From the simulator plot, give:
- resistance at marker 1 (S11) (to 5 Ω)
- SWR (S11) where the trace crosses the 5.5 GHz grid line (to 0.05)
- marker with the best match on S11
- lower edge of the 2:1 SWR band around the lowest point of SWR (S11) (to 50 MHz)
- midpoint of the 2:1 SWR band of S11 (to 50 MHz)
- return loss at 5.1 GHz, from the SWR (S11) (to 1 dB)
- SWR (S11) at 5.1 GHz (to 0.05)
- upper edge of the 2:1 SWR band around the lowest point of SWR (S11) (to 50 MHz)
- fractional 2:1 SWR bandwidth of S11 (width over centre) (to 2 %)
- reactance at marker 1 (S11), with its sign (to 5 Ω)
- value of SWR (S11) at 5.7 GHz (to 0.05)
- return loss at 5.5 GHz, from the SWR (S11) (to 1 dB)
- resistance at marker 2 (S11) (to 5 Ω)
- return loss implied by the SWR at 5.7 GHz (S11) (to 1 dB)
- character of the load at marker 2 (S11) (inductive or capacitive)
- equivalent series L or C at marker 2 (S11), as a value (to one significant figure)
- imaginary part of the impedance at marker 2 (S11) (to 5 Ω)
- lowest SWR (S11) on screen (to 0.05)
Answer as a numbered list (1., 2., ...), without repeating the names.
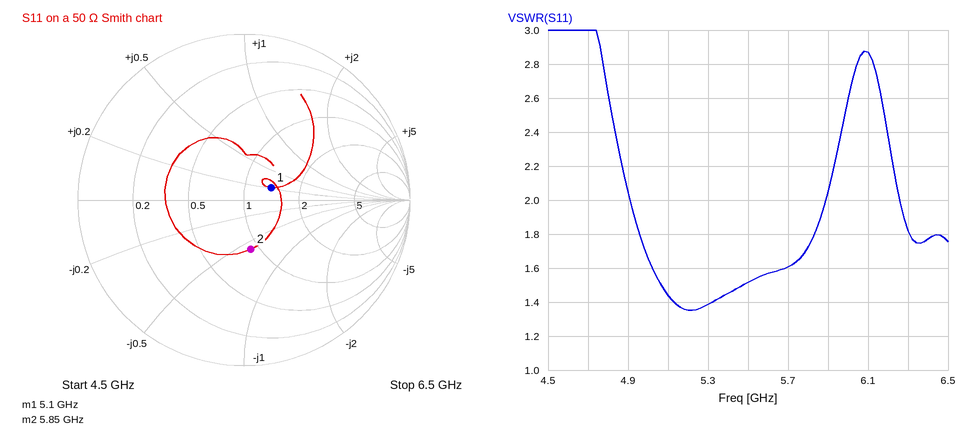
1. 70 Ω
2. 1.50
3. marker 1
4. 4.90 GHz
5. 5.40 GHz
6. 15 dB
7. 1.45
8. 5.90 GHz
9. 18 %
10. +10 Ω
11. 1.60
12. 14 dB
13. 45 Ω
14. 13 dB
15. capacitive
16. 900 fF
17. -30 Ω
18. 1.35
